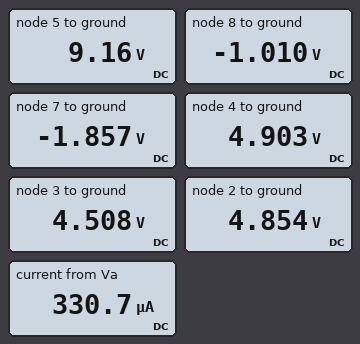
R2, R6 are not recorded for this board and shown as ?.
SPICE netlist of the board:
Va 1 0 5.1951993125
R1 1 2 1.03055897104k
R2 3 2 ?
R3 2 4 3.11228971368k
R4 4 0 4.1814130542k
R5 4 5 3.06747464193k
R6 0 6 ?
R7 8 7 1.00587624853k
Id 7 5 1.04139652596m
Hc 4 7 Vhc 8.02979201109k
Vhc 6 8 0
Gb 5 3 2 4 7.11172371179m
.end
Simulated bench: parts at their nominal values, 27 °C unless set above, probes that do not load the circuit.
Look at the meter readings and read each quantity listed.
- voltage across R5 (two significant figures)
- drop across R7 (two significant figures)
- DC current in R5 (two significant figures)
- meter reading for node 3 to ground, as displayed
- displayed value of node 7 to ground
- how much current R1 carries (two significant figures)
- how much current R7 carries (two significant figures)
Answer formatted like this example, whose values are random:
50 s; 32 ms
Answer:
4.3 V; 850 mV; 1.4 mA; 4.508 V; -1.857 V; 330 µA; 840 µA
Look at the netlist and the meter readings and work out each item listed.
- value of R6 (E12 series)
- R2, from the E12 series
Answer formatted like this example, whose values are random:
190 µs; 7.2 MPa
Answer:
1.2 kΩ; 1 kΩ
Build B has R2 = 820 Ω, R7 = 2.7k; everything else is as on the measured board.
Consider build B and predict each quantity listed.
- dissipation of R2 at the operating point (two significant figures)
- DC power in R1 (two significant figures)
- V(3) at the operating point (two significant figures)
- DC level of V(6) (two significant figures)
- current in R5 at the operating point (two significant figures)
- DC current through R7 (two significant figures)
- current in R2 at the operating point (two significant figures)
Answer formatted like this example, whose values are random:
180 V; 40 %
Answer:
220 nW; 250 nW; 5.2 V; -1.5 V; 1.0 mA; 1.3 mA; 16 µA
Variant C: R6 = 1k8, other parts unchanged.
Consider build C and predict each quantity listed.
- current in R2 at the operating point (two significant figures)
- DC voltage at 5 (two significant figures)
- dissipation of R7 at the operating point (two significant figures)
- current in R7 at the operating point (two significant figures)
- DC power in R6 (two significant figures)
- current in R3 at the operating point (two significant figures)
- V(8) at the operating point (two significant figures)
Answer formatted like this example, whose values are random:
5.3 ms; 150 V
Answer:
250 µA; 8.9 V; 920 µW; 950 µA; 1.6 mW; 11 µA; -1.7 V
